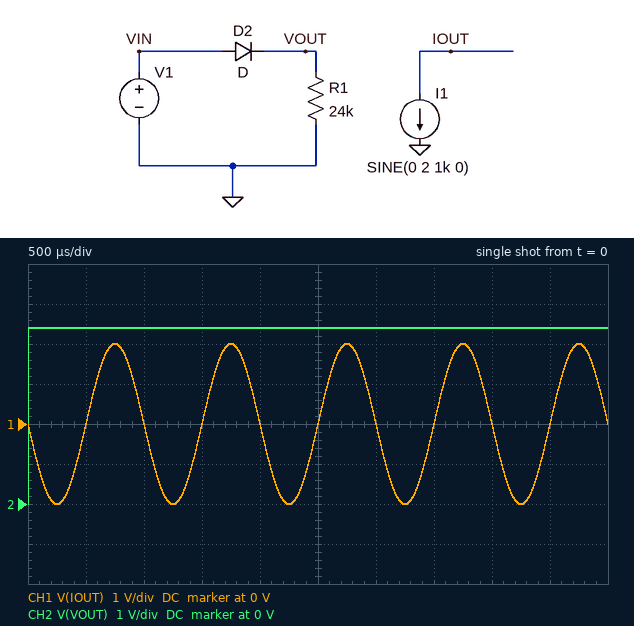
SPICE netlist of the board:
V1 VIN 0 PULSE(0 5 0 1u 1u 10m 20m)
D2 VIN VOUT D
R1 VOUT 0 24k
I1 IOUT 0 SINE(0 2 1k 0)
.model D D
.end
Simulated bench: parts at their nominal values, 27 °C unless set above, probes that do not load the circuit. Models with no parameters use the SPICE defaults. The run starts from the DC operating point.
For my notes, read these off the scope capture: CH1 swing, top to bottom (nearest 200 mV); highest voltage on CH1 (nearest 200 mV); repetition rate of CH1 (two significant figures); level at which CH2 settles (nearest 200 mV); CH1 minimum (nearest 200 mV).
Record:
4.0 V
2.0 V
1.0 kHz
4.4 V
-2.0 V
